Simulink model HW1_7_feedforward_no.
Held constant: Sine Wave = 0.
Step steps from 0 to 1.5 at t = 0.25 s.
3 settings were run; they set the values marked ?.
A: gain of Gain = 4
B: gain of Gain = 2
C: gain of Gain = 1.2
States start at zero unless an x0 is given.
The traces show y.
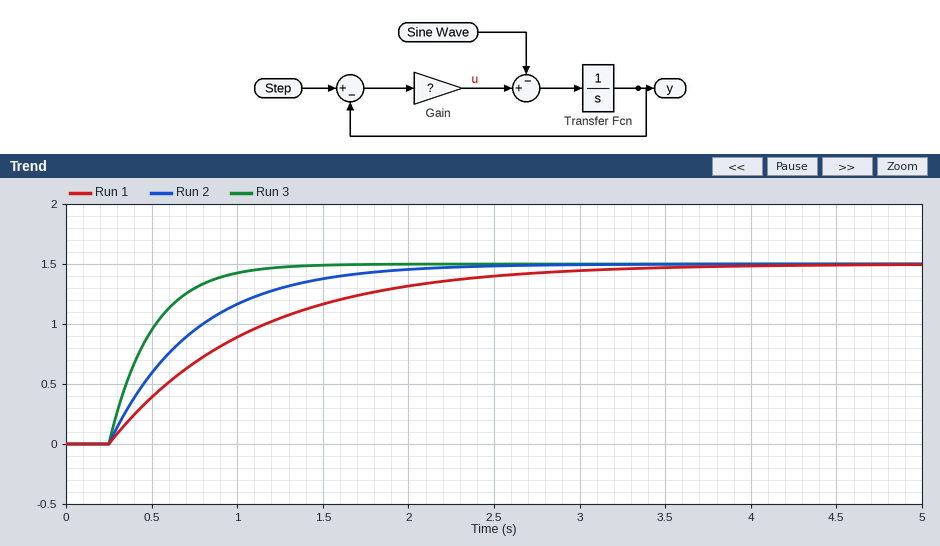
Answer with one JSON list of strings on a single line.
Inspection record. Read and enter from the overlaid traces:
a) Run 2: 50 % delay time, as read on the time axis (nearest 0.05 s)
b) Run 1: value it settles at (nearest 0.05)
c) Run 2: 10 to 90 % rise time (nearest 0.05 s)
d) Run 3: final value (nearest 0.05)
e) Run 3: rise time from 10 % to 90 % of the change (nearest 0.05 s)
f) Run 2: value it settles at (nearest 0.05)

["0.60 s", "1.50", "1.10 s", "1.50", "0.55 s", "1.50"]
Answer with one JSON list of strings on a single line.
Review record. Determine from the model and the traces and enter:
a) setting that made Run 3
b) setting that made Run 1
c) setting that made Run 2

["A", "C", "B"]
